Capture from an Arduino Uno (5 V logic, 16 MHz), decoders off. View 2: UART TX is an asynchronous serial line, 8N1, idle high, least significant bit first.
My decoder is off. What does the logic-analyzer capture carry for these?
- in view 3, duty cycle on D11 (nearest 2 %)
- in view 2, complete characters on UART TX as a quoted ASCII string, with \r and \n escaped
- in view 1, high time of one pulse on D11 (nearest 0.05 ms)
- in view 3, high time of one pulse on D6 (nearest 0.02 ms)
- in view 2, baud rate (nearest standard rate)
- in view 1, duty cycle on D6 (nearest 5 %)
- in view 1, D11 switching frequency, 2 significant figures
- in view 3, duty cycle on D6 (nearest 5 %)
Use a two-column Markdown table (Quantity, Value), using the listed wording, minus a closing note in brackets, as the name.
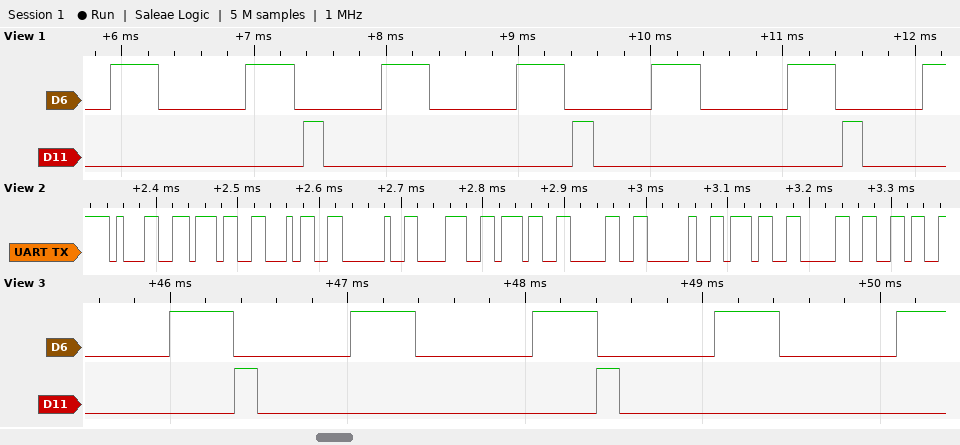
| Quantity | Value |
|---|---|
| in view 3, duty cycle on D11 | 6 % |
| in view 2, complete characters on UART TX as a quoted ASCII string, with \r and \n escaped | "174 870 706" |
| in view 1, high time of one pulse on D11 | 0.15 ms |
| in view 3, high time of one pulse on D6 | 0.36 ms |
| in view 2, baud rate | 115200 baud |
| in view 1, duty cycle on D6 | 35 % |
| in view 1, D11 switching frequency, 2 significant figures | 490 Hz |
| in view 3, duty cycle on D6 | 35 % |
